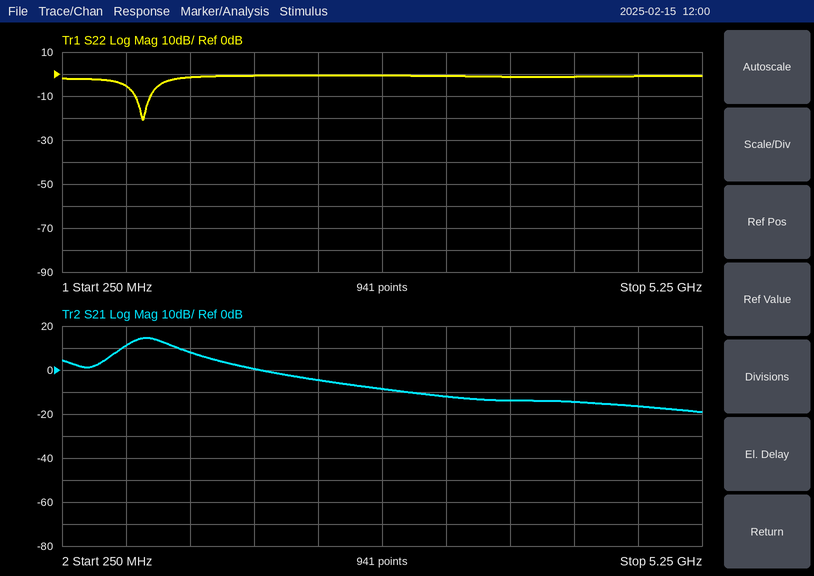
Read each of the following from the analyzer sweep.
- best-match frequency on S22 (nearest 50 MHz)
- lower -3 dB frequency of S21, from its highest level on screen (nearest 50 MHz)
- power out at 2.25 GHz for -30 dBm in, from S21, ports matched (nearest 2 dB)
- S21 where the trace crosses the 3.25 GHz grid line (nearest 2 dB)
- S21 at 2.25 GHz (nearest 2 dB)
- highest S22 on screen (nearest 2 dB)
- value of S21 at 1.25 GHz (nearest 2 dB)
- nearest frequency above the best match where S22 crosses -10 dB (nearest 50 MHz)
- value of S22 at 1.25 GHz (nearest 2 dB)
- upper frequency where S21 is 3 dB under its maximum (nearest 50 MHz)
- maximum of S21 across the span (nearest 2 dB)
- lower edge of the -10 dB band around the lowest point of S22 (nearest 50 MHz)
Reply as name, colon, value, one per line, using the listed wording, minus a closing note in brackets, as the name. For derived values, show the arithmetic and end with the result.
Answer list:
best-match frequency on S22: 900 MHz
lower -3 dB frequency of S21, from its highest level on screen: 750 MHz
power out at 2.25 GHz for -30 dBm in, from S21, ports matched: -30 dBm + (-4 dB) = -34 dBm
S21 where the trace crosses the 3.25 GHz grid line: -12 dB
S21 at 2.25 GHz: -4 dB
highest S22 on screen: 0 dB
value of S21 at 1.25 GHz: 8 dB
nearest frequency above the best match where S22 crosses -10 dB: 950 MHz
value of S22 at 1.25 GHz: -2 dB
upper frequency where S21 is 3 dB under its maximum: 1.10 GHz
maximum of S21 across the span: 14 dB
lower edge of the -10 dB band around the lowest point of S22: 800 MHz
